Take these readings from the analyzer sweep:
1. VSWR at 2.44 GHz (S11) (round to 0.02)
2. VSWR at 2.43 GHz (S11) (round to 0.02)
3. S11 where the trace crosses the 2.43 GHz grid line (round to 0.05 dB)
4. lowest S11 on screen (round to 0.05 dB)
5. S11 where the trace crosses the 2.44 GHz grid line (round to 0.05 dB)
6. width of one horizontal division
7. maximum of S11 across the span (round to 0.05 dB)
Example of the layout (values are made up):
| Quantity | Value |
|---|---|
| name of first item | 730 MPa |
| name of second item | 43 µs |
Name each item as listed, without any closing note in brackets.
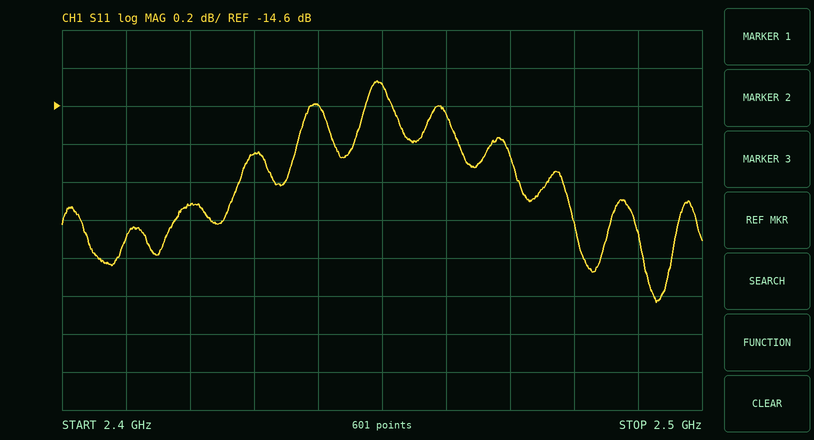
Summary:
| Quantity | Value |
|---|---|
| VSWR at 2.44 GHz (S11) | 1.46 |
| VSWR at 2.43 GHz (S11) | 1.44 |
| S11 where the trace crosses the 2.43 GHz grid line | -14.85 dB |
| lowest S11 on screen | -15.65 dB |
| S11 where the trace crosses the 2.44 GHz grid line | -14.60 dB |
| width of one horizontal division | 10 MHz |
| maximum of S11 across the span | -14.45 dB |
